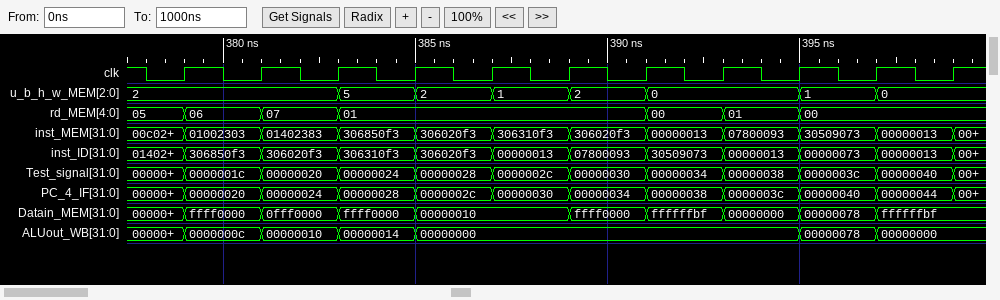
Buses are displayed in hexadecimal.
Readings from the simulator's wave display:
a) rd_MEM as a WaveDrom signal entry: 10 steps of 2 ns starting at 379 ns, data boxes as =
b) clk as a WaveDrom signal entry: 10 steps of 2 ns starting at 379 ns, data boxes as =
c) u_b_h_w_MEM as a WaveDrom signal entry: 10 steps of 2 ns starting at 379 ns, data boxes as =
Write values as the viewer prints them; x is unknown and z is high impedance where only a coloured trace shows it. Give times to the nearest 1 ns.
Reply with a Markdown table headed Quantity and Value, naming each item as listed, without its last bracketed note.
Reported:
| Quantity | Value |
|---|---|
| rd_MEM as a WaveDrom signal entry: 10 steps of 2 ns starting at 379 ns, data boxes as = | {name: 'rd_MEM', wave: '===...===.', data: '06 07 01 00 01 00'} |
| clk as a WaveDrom signal entry: 10 steps of 2 ns starting at 379 ns, data boxes as = | {name: 'clk', wave: 'p.........'} |
| u_b_h_w_MEM as a WaveDrom signal entry: 10 steps of 2 ns starting at 379 ns, data boxes as = | {name: 'u_b_h_w_MEM', wave: '=.=====.==', data: '2 5 2 1 2 0 1 0'} |
